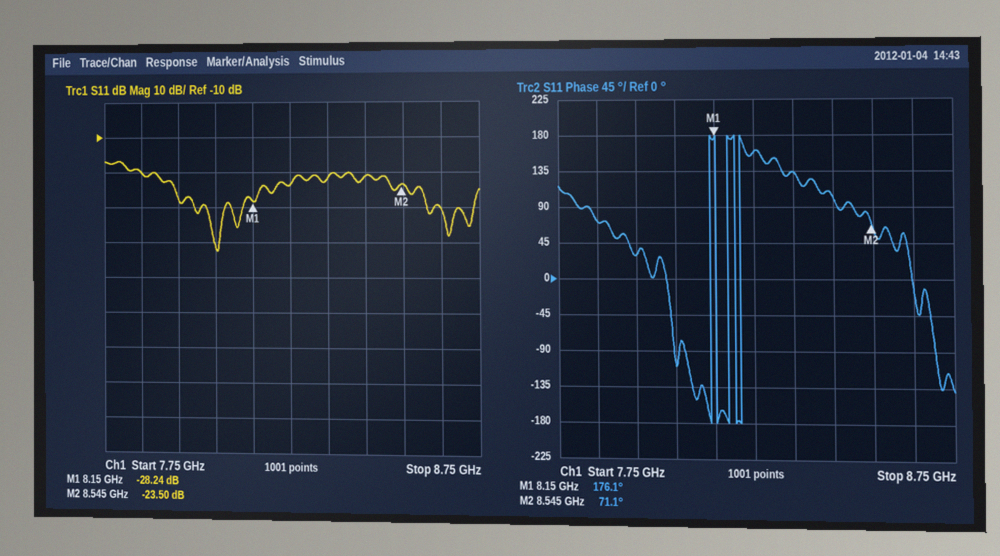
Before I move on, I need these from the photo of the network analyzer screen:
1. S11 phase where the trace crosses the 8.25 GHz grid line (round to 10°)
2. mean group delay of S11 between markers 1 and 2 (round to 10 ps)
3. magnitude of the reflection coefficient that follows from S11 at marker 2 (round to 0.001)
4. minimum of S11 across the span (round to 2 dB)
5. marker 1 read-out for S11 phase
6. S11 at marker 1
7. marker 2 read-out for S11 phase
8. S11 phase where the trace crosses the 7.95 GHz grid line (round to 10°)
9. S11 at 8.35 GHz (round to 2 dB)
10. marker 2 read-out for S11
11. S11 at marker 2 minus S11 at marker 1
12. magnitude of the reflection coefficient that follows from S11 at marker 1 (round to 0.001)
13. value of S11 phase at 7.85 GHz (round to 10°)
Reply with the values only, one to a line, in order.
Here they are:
160°
740 ps
0.067
-42 dB
176.1°
-28.24 dB
71.1°
30°
-22 dB
-23.50 dB
4.74 dB
0.039
70°
